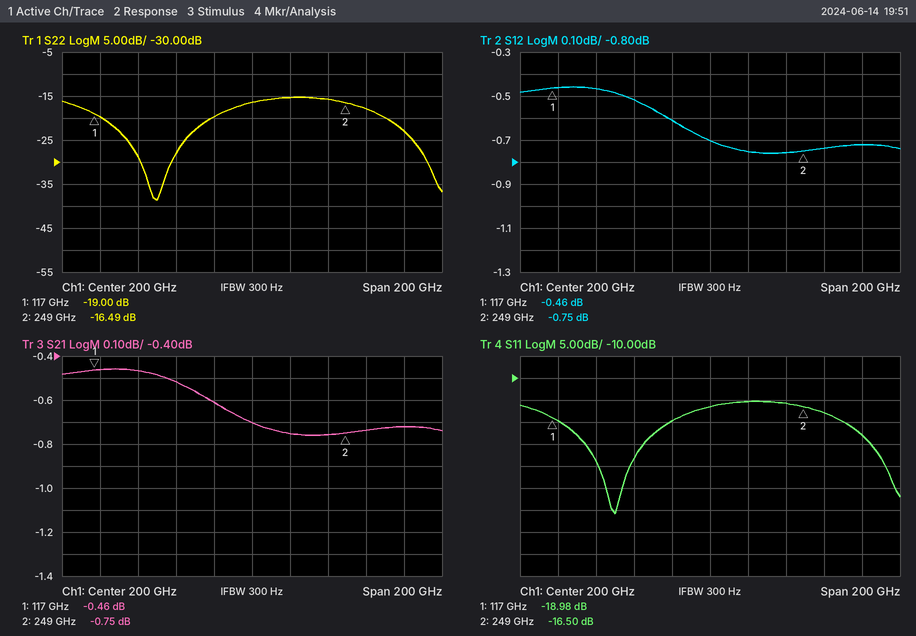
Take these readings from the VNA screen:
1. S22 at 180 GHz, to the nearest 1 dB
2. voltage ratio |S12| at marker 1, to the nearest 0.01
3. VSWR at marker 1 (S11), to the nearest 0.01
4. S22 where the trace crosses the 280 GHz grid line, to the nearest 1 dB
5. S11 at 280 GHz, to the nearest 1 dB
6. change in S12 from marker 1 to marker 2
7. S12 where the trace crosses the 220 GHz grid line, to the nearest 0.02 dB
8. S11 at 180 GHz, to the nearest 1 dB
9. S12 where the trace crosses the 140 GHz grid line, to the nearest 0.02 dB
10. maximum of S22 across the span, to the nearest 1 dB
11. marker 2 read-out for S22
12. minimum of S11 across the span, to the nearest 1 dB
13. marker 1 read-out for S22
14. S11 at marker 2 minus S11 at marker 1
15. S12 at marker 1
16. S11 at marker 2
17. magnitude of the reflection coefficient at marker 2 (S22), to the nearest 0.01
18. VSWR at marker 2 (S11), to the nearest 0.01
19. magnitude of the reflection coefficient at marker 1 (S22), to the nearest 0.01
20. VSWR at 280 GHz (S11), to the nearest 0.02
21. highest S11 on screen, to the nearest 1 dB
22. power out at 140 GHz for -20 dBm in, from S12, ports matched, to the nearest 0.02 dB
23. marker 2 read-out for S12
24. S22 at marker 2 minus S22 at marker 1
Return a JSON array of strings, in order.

["-20 dB", "0.95", "1.25", "-23 dB", "-23 dB", "-0.29 dB", "-0.76 dB", "-20 dB", "-0.46 dB", "-15 dB", "-16.49 dB", "-41 dB", "-19.00 dB", "2.48 dB", "-0.46 dB", "-16.50 dB", "0.15", "1.35", "0.11", "1.16", "-15 dB", "-20.46 dBm", "-0.75 dB", "2.51 dB"]
